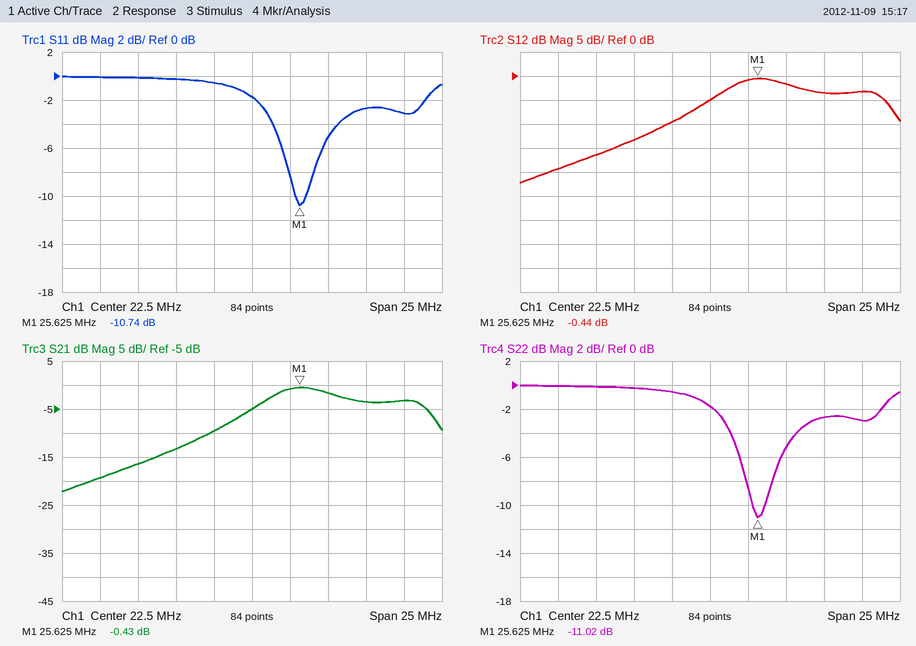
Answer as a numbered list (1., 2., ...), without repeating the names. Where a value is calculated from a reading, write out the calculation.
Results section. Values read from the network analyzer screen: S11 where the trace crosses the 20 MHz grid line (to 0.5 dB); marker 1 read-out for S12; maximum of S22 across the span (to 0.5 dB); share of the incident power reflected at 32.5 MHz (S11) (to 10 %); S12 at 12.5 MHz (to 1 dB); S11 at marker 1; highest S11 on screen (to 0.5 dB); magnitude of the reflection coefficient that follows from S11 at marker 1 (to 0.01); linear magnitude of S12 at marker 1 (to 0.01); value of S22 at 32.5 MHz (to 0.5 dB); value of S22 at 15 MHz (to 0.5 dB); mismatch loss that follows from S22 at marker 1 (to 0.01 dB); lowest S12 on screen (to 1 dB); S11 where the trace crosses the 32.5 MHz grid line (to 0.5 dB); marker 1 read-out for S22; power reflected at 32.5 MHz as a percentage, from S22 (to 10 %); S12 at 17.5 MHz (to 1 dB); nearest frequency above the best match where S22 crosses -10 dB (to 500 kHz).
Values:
1. -0.5 dB
2. -0.44 dB
3. 0.0 dB
4. 10^(-3/10) ≈ 50 %
5. -19 dB
6. -10.74 dB
7. 0.0 dB
8. 10^(-10.74/20) ≈ 0.29
9. 10^(-0.44/20) ≈ 0.95
10. -3.0 dB
11. 0.0 dB
12. −10 log10(1 − 10^(-11.02/10)) ≈ 0.36 dB
13. -22 dB
14. -3.0 dB
15. -11.02 dB
16. 10^(-3/10) ≈ 50 %
17. -13 dB
18. 26.0 MHz
